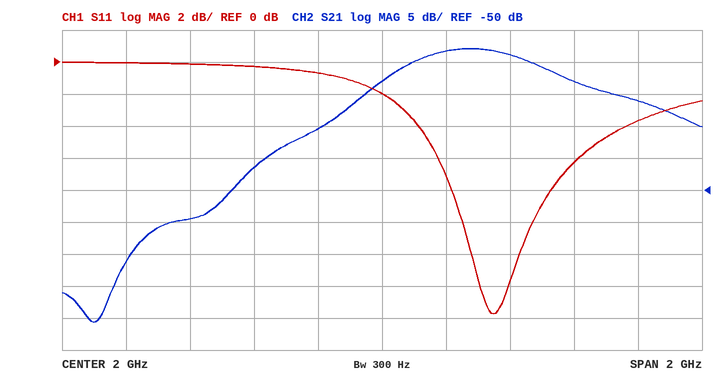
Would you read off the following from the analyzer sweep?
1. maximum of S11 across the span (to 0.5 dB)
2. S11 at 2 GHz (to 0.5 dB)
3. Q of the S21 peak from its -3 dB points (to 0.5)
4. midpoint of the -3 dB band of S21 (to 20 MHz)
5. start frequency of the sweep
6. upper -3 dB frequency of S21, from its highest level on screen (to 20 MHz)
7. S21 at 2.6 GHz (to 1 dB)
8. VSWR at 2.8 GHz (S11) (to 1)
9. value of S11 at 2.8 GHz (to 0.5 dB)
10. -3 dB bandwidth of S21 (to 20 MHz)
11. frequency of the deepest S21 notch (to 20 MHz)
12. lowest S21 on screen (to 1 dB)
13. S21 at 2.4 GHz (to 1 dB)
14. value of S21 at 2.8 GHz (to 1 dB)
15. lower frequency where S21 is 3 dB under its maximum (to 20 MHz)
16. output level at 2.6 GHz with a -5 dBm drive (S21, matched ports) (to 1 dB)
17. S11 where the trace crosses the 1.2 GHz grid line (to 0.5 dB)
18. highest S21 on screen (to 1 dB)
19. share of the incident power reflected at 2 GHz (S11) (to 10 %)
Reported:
0.0 dB
-2.0 dB
5.0
2.28 GHz
1 GHz
2.50 GHz
-33 dB
5
-3.5 dB
440 MHz
1.10 GHz
-71 dB
-29 dB
-36 dB
2.06 GHz
-38 dBm
0.0 dB
-28 dB
60 %
